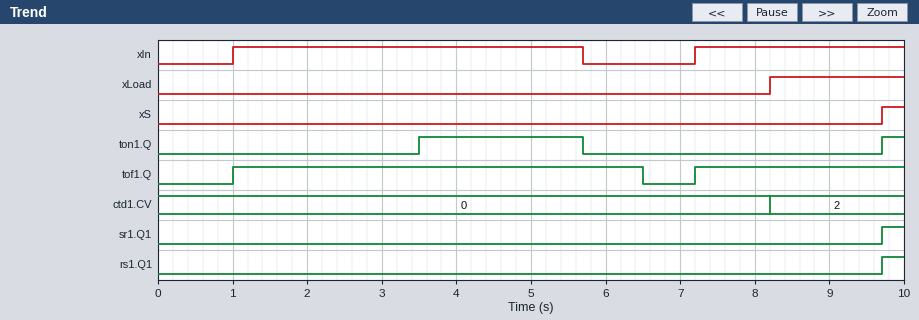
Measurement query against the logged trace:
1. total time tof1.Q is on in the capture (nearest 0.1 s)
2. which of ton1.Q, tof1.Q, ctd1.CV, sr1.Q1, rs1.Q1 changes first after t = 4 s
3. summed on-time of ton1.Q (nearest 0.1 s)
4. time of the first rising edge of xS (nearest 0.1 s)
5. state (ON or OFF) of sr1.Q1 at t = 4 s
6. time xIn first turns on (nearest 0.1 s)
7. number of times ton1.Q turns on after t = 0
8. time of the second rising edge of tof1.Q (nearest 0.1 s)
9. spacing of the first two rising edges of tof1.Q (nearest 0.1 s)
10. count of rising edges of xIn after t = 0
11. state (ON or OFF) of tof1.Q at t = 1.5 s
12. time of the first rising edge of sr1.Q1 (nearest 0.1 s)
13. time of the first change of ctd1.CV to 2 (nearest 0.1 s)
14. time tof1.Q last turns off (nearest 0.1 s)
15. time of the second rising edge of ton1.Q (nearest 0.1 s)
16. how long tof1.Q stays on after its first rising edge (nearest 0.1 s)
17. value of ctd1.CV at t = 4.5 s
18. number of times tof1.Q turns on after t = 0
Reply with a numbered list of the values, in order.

1. 8.3 s
2. ton1.Q
3. 2.5 s
4. 9.7 s
5. OFF
6. 1.0 s
7. 2
8. 7.2 s
9. 6.2 s
10. 2
11. ON
12. 9.7 s
13. 8.2 s
14. 6.5 s
15. 9.7 s
16. 5.5 s
17. 0
18. 2
